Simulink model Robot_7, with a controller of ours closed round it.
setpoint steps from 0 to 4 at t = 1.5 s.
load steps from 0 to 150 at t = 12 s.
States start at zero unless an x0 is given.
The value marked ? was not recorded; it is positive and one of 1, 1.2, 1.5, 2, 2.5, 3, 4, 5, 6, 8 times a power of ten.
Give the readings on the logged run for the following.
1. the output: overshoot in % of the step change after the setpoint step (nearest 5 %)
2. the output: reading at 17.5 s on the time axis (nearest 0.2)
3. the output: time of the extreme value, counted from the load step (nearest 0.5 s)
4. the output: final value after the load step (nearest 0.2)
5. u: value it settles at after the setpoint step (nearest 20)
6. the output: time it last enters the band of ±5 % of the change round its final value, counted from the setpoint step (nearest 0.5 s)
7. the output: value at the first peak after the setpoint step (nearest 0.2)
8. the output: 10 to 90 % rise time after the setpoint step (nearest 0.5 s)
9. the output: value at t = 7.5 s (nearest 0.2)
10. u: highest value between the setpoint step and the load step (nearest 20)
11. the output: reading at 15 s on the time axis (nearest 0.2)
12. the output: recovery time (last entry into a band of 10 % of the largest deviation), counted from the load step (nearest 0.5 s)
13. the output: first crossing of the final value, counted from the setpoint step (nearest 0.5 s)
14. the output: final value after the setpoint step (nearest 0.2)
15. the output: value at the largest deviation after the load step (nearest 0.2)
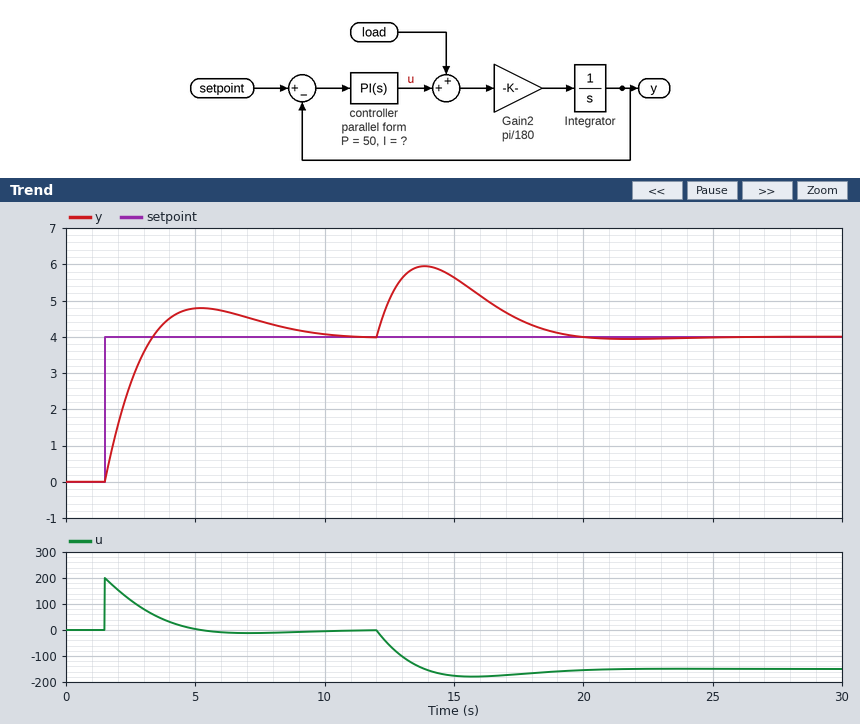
20 %
4.4
2.0 s
4.0
0
7.5 s
4.8
1.5 s
4.4
200
5.6
6.5 s
2.0 s
4.0
6.0
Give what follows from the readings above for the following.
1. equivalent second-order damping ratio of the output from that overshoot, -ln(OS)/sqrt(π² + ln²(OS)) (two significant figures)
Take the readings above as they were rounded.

0.46
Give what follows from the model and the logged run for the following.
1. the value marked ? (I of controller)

20
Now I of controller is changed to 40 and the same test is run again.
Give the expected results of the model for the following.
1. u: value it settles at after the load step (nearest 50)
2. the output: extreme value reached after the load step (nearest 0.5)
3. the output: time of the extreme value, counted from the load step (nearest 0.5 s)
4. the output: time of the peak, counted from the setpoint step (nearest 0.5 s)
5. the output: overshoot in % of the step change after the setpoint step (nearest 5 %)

-150
5.5
1.5 s
3.0 s
30 %
